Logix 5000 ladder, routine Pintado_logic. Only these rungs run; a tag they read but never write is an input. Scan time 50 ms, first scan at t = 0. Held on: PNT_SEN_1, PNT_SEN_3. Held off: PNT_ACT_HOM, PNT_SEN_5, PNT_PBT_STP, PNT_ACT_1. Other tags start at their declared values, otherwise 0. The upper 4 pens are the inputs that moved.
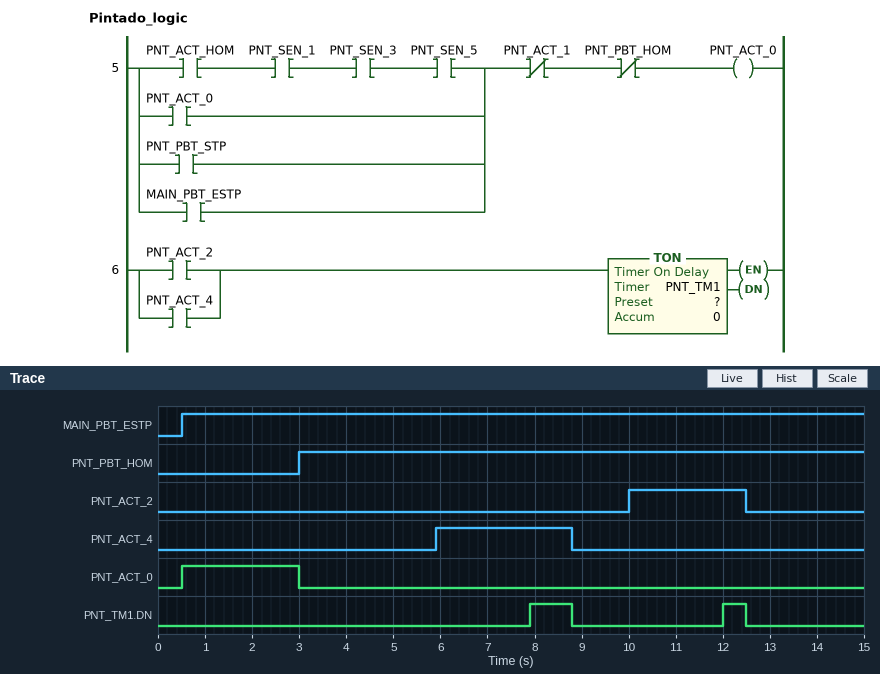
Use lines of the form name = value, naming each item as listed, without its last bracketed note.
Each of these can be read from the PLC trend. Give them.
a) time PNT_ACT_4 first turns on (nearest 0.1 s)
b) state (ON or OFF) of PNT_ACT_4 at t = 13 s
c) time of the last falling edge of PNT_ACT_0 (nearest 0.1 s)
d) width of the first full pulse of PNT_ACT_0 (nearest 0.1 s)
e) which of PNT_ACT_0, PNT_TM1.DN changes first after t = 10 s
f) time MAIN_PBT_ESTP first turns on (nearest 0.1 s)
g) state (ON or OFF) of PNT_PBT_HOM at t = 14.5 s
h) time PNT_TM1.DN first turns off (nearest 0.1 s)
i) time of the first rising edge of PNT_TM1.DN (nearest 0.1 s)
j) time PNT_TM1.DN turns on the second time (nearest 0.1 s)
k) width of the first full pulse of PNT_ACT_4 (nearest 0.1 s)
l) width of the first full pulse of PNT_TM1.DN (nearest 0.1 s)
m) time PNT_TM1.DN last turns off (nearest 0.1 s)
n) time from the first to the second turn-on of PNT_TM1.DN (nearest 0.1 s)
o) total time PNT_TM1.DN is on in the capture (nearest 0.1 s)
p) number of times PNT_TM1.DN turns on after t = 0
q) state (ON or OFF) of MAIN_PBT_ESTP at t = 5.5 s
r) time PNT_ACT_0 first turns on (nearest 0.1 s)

time PNT_ACT_4 first turns on = 5.9 s
state (ON or OFF) of PNT_ACT_4 at t = 13 s = OFF
time of the last falling edge of PNT_ACT_0 = 3.0 s
width of the first full pulse of PNT_ACT_0 = 2.5 s
which of PNT_ACT_0, PNT_TM1.DN changes first after t = 10 s = PNT_TM1.DN
time MAIN_PBT_ESTP first turns on = 0.5 s
state (ON or OFF) of PNT_PBT_HOM at t = 14.5 s = ON
time PNT_TM1.DN first turns off = 8.8 s
time of the first rising edge of PNT_TM1.DN = 7.9 s
time PNT_TM1.DN turns on the second time = 12.0 s
width of the first full pulse of PNT_ACT_4 = 2.9 s
width of the first full pulse of PNT_TM1.DN = 0.9 s
time PNT_TM1.DN last turns off = 12.5 s
time from the first to the second turn-on of PNT_TM1.DN = 4.1 s
total time PNT_TM1.DN is on in the capture = 1.4 s
number of times PNT_TM1.DN turns on after t = 0 = 2
state (ON or OFF) of MAIN_PBT_ESTP at t = 5.5 s = ON
time PNT_ACT_0 first turns on = 0.5 s
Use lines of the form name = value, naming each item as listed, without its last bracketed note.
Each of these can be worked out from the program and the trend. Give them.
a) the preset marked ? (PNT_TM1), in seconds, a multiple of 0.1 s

the preset marked ? (PNT_TM1), in seconds, a multiple of 0.1 s = 2.0 s
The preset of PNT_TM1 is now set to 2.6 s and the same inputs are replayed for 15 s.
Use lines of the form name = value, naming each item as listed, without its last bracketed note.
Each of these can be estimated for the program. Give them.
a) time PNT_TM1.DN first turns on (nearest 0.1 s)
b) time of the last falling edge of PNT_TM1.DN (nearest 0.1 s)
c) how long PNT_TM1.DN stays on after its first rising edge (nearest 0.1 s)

time PNT_TM1.DN first turns on = 8.5 s
time of the last falling edge of PNT_TM1.DN = 8.8 s
how long PNT_TM1.DN stays on after its first rising edge = 0.3 s
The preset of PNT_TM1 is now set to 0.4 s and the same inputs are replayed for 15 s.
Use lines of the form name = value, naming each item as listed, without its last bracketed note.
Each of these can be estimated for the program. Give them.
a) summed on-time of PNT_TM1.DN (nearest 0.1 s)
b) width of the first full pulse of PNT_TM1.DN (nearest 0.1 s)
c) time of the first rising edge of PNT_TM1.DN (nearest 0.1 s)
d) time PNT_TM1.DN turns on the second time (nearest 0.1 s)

summed on-time of PNT_TM1.DN = 4.6 s
width of the first full pulse of PNT_TM1.DN = 2.5 s
time of the first rising edge of PNT_TM1.DN = 6.3 s
time PNT_TM1.DN turns on the second time = 10.4 s
